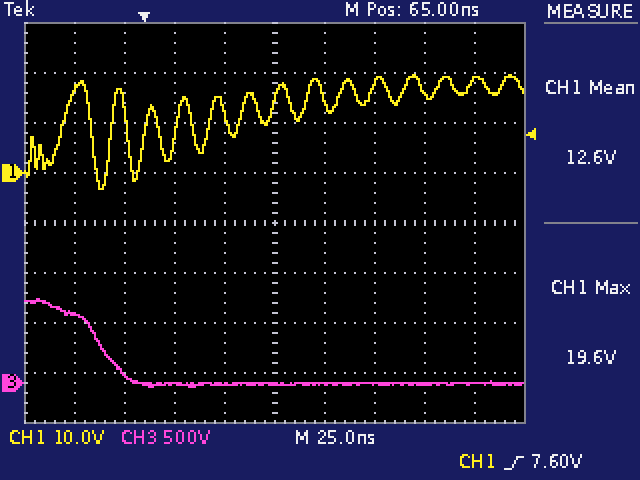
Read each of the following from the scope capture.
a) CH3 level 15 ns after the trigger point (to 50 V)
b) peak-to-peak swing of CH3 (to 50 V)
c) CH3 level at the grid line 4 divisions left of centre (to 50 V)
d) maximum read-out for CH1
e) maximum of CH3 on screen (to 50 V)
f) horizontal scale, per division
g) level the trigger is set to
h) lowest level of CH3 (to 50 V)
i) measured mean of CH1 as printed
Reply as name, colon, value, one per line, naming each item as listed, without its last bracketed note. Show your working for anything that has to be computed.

CH3 level 15 ns after the trigger point: 0 V
peak-to-peak swing of CH3: 850 V − (-50 V) = 900 V
CH3 level at the grid line 4 divisions left of centre: 700 V
maximum read-out for CH1: 19.6 V
maximum of CH3 on screen: 850 V
horizontal scale, per division: 25 ns
level the trigger is set to: 7.60 V
lowest level of CH3: -50 V
measured mean of CH1 as printed: 12.6 V
